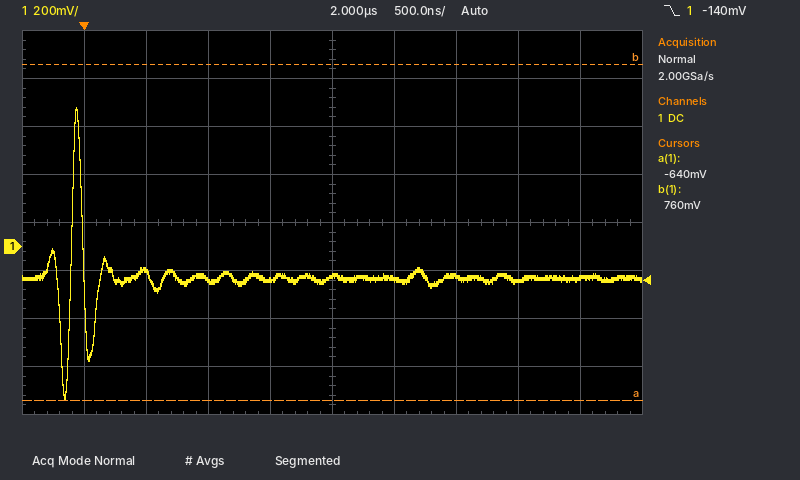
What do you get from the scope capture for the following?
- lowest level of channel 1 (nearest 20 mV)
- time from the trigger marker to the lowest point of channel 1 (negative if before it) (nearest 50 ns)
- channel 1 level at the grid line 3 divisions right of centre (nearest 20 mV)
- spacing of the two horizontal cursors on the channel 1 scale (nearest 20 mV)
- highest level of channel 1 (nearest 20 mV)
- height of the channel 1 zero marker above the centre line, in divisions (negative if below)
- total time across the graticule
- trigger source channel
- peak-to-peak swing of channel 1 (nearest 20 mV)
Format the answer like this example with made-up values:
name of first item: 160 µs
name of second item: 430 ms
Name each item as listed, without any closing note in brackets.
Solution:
lowest level of channel 1: -640 mV
time from the trigger marker to the lowest point of channel 1 (negative if before it): -150 ns
channel 1 level at the grid line 3 divisions right of centre: -140 mV
spacing of the two horizontal cursors on the channel 1 scale: 1.40 V
highest level of channel 1: 580 mV
height of the channel 1 zero marker above the centre line, in divisions: -0.5 div
total time across the graticule: 5 µs
trigger source channel: channel 1
peak-to-peak swing of channel 1: 1.22 V
